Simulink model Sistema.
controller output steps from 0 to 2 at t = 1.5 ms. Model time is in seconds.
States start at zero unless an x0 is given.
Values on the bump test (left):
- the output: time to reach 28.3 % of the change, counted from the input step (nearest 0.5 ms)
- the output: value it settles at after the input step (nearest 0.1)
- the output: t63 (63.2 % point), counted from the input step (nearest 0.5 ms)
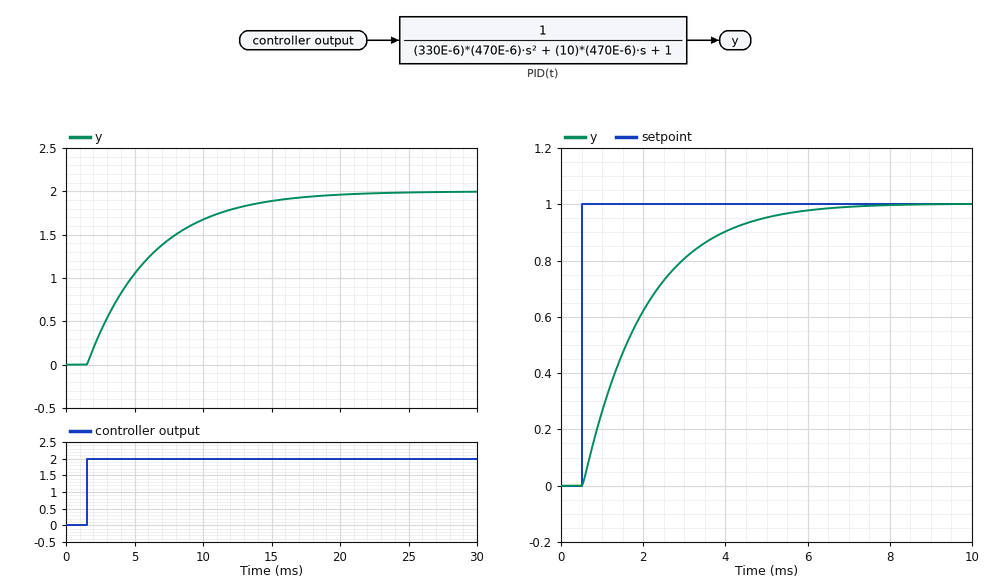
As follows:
1.5 ms
2.0
4.5 ms
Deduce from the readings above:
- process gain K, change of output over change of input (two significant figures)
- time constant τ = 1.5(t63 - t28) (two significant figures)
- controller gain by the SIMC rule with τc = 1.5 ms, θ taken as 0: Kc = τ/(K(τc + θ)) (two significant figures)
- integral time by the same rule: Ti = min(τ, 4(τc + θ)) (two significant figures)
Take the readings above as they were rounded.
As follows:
1.0
4.5 ms
3.0
4.5 ms
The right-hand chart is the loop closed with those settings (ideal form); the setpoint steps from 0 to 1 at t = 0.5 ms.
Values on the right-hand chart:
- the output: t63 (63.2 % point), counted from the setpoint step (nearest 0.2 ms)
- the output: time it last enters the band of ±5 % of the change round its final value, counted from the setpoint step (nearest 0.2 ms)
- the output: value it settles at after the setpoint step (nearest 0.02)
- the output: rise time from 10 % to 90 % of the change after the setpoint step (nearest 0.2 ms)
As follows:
1.6 ms
4.4 ms
1.00
3.2 ms
